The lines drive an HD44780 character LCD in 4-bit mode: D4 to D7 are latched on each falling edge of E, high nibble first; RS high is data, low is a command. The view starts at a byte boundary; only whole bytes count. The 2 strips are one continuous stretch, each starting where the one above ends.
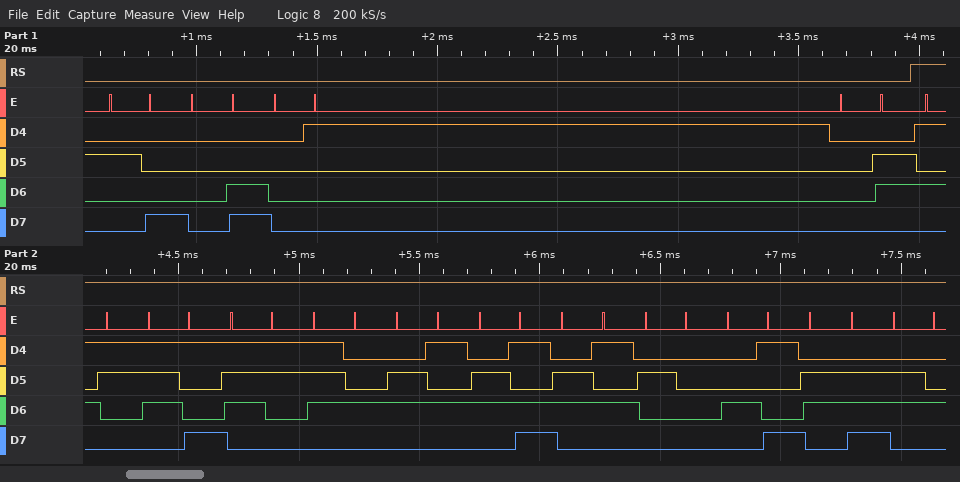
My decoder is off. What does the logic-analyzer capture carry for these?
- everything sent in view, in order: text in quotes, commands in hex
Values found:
0x28 0x0C 0x01 0x06 "Systeme Ind"
